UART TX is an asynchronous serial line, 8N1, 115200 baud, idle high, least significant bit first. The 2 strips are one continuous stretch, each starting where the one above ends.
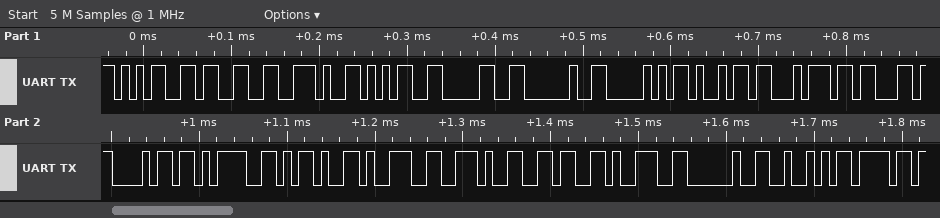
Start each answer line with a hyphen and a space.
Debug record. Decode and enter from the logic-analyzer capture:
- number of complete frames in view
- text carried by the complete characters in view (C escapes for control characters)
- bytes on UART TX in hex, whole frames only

- 20
- "53.50 Pitch=-9.69 Ro"
- 35 33 2E 35 30 20 50 69 74 63 68 3D 2D 39 2E 36 39 20 52 6F
